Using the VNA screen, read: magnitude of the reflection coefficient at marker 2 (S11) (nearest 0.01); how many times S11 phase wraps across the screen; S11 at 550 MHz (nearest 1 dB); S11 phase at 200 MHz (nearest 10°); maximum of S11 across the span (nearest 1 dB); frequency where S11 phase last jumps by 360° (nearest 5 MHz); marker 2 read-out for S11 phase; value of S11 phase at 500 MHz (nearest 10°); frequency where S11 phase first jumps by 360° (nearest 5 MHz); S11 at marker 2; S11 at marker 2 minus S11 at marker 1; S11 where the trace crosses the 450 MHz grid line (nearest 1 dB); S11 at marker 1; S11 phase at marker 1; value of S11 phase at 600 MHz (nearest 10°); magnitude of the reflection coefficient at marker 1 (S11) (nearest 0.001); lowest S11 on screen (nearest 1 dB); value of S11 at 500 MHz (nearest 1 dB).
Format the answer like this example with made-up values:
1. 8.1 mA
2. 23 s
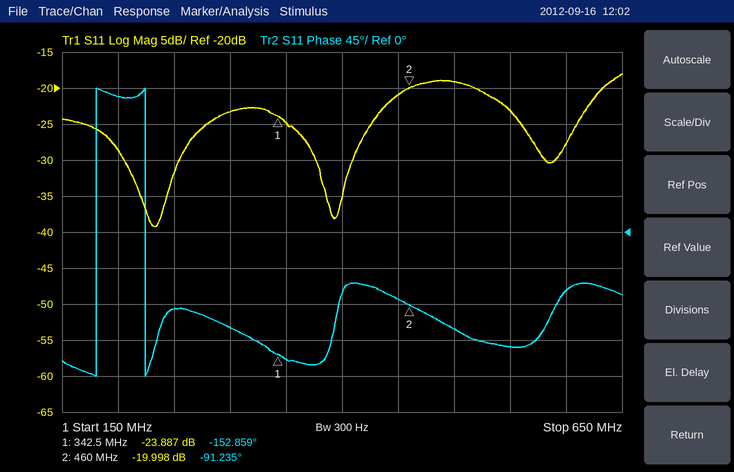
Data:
1. 0.10
2. 2
3. -23 dB
4. 170°
5. -18 dB
6. 225 MHz
7. -91.235°
8. -120°
9. 180 MHz
10. -19.998 dB
11. 3.889 dB
12. -21 dB
13. -23.887 dB
14. -152.859°
15. -70°
16. 0.064
17. -39 dB
18. -19 dB
